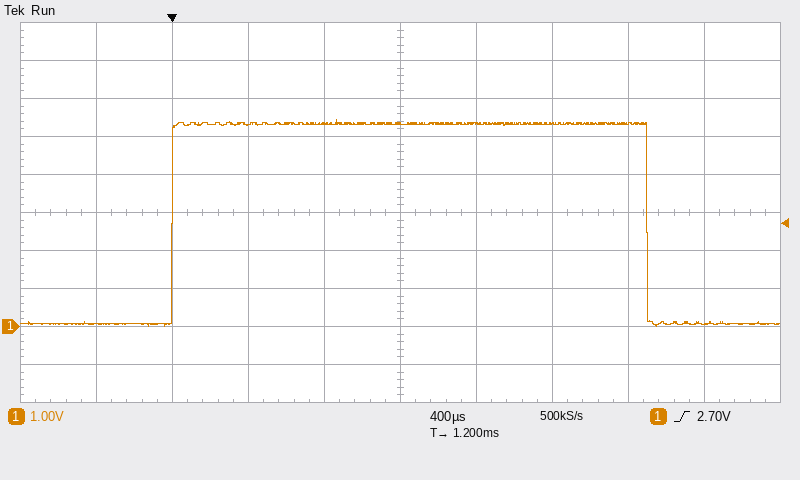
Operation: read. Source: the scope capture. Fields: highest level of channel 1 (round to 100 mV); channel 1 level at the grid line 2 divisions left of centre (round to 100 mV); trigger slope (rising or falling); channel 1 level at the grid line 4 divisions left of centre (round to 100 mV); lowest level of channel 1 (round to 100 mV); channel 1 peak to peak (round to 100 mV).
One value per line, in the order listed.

5.4 V
5.3 V
rising
100 mV
0.0 V
5.4 V
